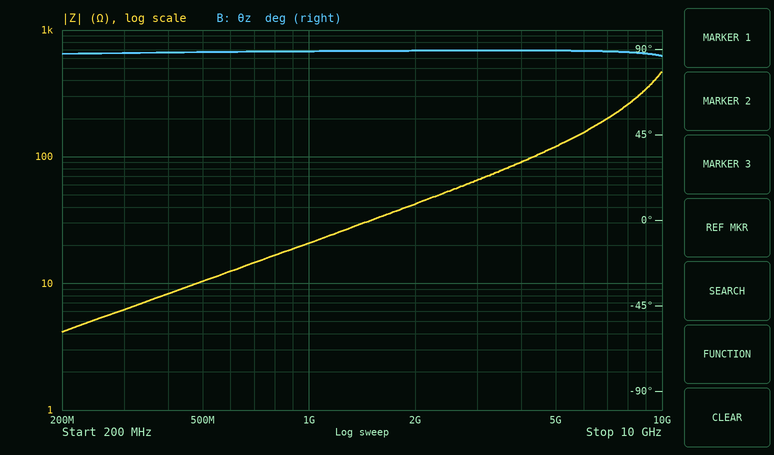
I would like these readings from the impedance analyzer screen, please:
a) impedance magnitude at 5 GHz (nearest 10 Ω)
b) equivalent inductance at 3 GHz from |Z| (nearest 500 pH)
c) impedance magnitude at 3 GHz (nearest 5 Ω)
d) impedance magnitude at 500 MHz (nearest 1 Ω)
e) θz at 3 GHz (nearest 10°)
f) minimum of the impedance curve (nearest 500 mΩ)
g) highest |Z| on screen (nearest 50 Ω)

120 Ω
3.5 nH
65 Ω
10 Ω
90°
4.0 Ω
450 Ω
